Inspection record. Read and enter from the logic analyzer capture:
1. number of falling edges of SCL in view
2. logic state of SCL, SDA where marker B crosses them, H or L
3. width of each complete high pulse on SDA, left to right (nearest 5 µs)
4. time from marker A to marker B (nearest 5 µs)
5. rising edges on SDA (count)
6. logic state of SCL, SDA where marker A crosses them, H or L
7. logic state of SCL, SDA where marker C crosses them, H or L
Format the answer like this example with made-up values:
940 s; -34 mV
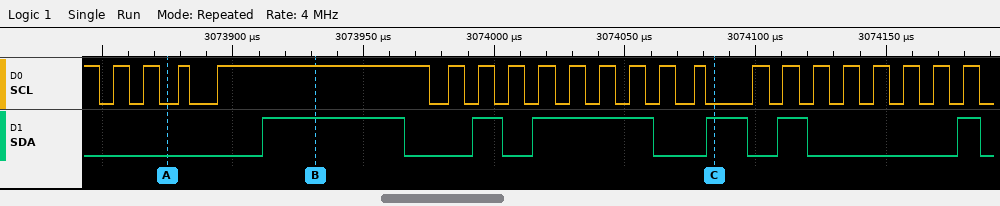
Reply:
22; SCL=H, SDA=H; 55 µs, 10 µs, 45 µs, 15 µs, 10 µs, 10 µs; 55 µs; 6; SCL=L, SDA=L; SCL=L, SDA=H
